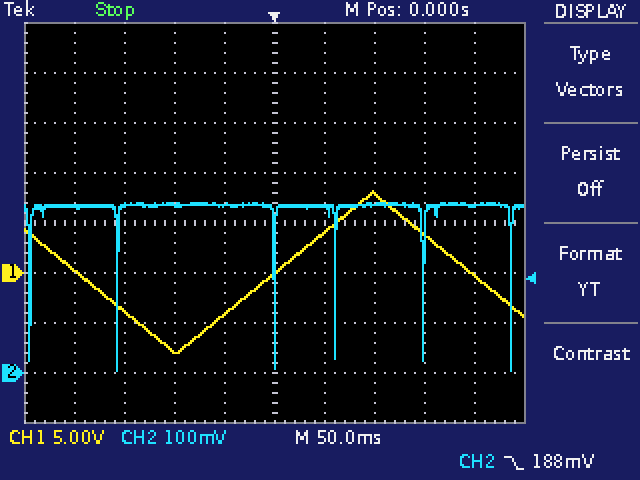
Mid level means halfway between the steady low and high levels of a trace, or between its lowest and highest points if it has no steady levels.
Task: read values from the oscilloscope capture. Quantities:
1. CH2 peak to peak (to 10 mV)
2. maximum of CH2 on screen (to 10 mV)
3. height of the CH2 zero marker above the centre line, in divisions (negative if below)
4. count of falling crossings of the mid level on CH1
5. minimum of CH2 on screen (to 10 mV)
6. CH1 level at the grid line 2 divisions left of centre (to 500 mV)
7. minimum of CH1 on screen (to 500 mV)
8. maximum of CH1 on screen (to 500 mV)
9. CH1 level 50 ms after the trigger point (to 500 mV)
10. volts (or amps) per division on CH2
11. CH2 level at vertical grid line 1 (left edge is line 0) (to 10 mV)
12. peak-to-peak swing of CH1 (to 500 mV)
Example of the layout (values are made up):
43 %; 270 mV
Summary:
340 mV; 340 mV; -3.0 div; 2; 0 mV; -8.0 V; -8.0 V; 8.0 V; 4.0 V; 100 mV; 330 mV; 16.0 V
